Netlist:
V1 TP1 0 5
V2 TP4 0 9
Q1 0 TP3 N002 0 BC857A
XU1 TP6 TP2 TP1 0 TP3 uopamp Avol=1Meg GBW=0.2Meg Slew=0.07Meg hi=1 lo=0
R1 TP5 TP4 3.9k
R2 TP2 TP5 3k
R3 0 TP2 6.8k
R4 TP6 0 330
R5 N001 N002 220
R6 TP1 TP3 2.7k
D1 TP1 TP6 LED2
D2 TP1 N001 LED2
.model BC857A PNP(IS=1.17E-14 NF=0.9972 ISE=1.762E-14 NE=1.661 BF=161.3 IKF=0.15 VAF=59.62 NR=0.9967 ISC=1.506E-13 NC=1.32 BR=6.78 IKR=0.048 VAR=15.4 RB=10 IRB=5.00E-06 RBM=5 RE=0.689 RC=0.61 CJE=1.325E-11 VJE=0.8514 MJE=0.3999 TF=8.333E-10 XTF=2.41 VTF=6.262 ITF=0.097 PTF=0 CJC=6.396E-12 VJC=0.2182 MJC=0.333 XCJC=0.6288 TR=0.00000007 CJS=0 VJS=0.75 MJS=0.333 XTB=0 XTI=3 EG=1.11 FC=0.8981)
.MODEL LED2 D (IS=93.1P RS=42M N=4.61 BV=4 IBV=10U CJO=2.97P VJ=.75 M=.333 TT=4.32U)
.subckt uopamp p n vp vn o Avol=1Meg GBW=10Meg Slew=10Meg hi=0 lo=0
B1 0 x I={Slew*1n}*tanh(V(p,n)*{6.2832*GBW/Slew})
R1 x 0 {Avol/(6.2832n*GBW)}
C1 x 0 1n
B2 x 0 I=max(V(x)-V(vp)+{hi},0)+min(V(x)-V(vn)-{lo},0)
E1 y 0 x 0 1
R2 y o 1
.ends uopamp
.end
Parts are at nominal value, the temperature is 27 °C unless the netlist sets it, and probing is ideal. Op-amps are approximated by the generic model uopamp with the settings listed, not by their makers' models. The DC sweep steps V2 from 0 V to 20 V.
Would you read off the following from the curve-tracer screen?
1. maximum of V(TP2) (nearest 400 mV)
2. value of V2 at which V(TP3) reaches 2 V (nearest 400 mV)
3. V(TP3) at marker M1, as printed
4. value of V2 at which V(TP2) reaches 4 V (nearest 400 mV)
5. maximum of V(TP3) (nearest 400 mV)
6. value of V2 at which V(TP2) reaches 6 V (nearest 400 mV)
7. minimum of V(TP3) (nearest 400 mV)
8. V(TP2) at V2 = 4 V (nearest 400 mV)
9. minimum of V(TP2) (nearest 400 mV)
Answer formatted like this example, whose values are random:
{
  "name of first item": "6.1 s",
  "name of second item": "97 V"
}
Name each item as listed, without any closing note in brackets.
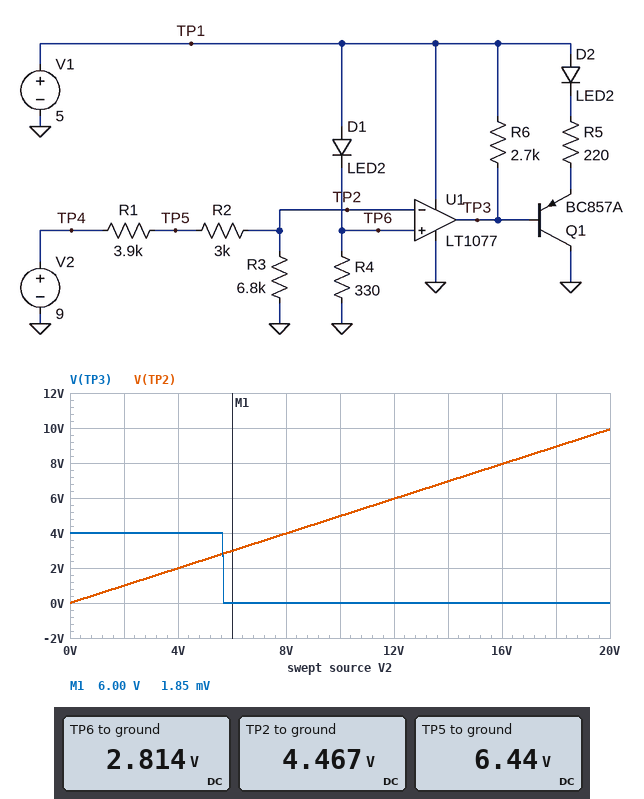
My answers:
{
  "maximum of V(TP2)": "10.0 V",
  "value of V2 at which V(TP3) reaches 2 V": "5.6 V",
  "V(TP3) at marker M1, as printed": "1.85 mV",
  "value of V2 at which V(TP2) reaches 4 V": "8.0 V",
  "maximum of V(TP3)": "4.0 V",
  "value of V2 at which V(TP2) reaches 6 V": "12.0 V",
  "minimum of V(TP3)": "0 V",
  "V(TP2) at V2 = 4 V": "2.0 V",
  "minimum of V(TP2)": "0 V"
}
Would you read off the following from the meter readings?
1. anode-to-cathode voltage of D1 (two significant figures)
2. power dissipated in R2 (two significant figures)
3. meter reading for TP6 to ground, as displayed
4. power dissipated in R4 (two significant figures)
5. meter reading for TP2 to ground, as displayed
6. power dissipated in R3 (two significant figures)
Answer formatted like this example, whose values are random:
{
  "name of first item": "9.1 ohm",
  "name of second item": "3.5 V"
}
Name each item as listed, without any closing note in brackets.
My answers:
{
  "anode-to-cathode voltage of D1": "2.2 V",
  "power dissipated in R2": "1.3 mW",
  "meter reading for TP6 to ground, as displayed": "2.814 V",
  "power dissipated in R4": "24 mW",
  "meter reading for TP2 to ground, as displayed": "4.467 V",
  "power dissipated in R3": "2.9 mW"
}
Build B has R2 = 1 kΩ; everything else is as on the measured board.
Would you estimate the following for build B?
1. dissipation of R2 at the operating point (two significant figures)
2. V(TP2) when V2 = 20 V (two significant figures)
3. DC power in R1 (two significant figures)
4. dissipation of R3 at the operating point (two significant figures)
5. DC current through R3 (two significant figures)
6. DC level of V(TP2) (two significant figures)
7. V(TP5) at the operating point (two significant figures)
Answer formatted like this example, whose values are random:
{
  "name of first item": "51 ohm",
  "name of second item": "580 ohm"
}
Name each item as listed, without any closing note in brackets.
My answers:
{
  "dissipation of R2 at the operating point": "590 µW",
  "V(TP2) when V2 = 20 V": "12 V",
  "DC power in R1": "2.3 mW",
  "dissipation of R3 at the operating point": "4.0 mW",
  "DC current through R3": "770 µA",
  "DC level of V(TP2)": "5.2 V",
  "V(TP5) at the operating point": "6.0 V"
}
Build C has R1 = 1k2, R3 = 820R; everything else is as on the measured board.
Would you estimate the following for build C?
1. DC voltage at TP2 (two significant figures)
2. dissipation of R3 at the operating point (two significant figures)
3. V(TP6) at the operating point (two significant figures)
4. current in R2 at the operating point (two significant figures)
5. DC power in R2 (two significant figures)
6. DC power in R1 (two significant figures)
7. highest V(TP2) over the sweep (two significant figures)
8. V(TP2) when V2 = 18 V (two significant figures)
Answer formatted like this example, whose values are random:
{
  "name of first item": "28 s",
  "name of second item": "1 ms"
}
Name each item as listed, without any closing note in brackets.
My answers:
{
  "DC voltage at TP2": "1.5 V",
  "dissipation of R3 at the operating point": "2.6 mW",
  "V(TP6) at the operating point": "2.8 V",
  "current in R2 at the operating point": "1.8 mA",
  "DC power in R2": "9.6 mW",
  "DC power in R1": "3.9 mW",
  "highest V(TP2) over the sweep": "3.3 V",
  "V(TP2) when V2 = 18 V": "2.9 V"
}
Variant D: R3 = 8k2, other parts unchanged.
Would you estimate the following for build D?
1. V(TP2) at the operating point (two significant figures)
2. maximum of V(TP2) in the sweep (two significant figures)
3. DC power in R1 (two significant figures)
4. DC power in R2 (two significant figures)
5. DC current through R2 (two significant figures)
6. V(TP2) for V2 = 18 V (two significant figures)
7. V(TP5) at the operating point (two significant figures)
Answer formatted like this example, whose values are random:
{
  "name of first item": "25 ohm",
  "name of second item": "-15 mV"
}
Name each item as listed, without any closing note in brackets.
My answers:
{
  "V(TP2) at the operating point": "4.9 V",
  "maximum of V(TP2) in the sweep": "11 V",
  "DC power in R1": "1.4 mW",
  "DC power in R2": "1.1 mW",
  "DC current through R2": "600 µA",
  "V(TP2) for V2 = 18 V": "9.8 V",
  "V(TP5) at the operating point": "6.7 V"
}
